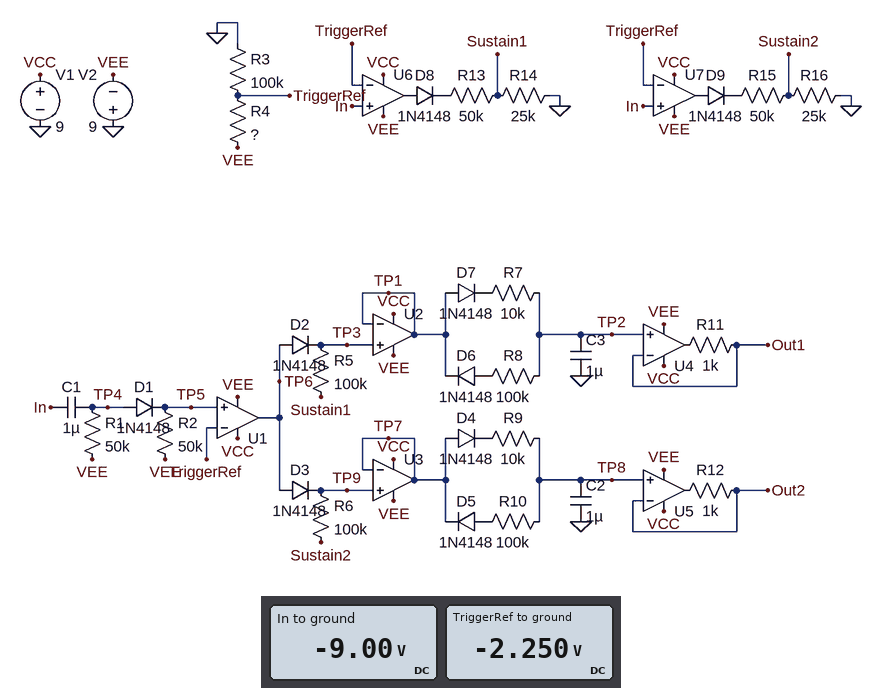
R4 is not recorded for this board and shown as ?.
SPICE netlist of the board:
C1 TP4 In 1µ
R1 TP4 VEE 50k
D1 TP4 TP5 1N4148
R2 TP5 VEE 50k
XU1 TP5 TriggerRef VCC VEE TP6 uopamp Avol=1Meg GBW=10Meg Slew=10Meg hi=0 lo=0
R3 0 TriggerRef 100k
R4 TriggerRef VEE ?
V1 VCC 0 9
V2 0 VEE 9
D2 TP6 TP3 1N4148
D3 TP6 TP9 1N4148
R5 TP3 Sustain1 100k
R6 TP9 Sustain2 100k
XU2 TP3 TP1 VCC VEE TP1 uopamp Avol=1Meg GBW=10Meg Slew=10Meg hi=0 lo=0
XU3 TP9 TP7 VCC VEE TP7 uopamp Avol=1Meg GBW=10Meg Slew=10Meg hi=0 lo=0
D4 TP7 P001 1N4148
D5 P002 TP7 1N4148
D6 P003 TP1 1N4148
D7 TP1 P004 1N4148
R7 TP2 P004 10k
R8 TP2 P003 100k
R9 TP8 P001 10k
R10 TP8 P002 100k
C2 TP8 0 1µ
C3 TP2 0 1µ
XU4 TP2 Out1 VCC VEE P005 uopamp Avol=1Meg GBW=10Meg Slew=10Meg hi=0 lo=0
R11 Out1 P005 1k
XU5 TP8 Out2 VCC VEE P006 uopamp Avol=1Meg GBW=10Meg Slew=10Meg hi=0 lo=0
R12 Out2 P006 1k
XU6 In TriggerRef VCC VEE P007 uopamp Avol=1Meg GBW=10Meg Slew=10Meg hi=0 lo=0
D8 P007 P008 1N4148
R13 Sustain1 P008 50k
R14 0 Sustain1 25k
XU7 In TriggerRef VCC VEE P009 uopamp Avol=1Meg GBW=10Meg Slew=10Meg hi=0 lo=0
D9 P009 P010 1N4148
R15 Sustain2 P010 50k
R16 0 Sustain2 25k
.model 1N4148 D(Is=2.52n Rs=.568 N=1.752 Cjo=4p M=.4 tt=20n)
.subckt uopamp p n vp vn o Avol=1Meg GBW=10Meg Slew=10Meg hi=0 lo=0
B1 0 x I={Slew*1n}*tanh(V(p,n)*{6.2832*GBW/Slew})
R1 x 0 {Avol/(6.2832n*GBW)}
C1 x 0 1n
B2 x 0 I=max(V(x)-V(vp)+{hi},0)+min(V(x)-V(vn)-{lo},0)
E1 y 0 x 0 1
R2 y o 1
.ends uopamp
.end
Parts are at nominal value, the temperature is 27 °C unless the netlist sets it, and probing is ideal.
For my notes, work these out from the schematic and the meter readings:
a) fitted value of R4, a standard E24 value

300 kΩ
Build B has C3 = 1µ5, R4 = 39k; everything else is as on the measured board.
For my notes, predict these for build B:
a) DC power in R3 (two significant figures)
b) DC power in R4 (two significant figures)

420 µW
160 µW
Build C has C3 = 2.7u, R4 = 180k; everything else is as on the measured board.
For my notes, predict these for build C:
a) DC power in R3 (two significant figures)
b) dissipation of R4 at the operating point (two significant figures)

100 µW
190 µW
